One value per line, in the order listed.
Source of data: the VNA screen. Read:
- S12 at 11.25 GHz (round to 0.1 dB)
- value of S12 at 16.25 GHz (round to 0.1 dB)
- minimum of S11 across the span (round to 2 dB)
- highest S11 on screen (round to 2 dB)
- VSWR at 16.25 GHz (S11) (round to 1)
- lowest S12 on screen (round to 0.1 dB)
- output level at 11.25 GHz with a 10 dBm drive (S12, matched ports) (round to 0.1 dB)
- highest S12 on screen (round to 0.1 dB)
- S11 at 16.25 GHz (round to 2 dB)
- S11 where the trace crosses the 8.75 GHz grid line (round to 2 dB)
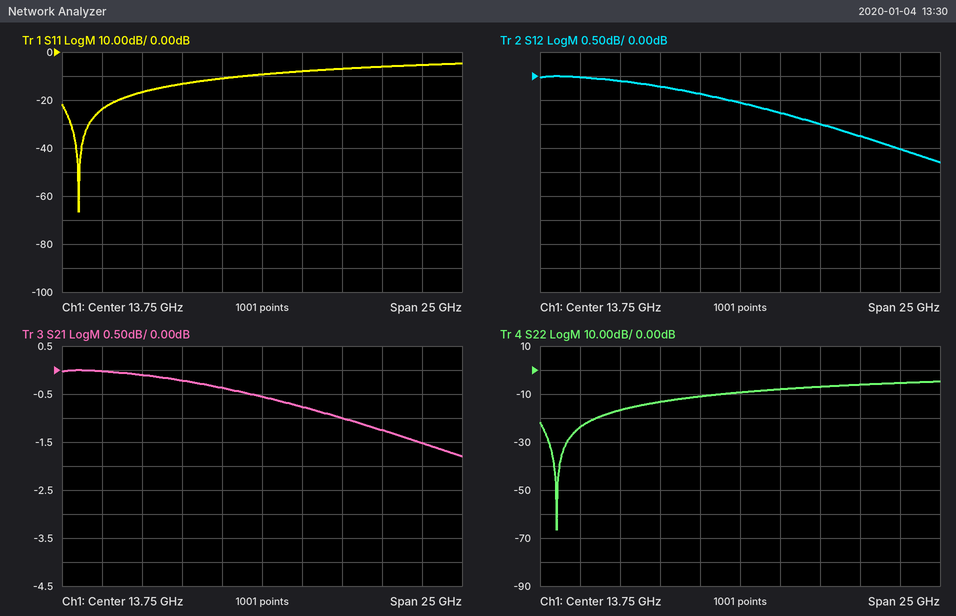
-0.4 dB
-0.8 dB
-66 dB
-4 dB
2
-1.8 dB
9.6 dBm
0.0 dB
-8 dB
-14 dB
